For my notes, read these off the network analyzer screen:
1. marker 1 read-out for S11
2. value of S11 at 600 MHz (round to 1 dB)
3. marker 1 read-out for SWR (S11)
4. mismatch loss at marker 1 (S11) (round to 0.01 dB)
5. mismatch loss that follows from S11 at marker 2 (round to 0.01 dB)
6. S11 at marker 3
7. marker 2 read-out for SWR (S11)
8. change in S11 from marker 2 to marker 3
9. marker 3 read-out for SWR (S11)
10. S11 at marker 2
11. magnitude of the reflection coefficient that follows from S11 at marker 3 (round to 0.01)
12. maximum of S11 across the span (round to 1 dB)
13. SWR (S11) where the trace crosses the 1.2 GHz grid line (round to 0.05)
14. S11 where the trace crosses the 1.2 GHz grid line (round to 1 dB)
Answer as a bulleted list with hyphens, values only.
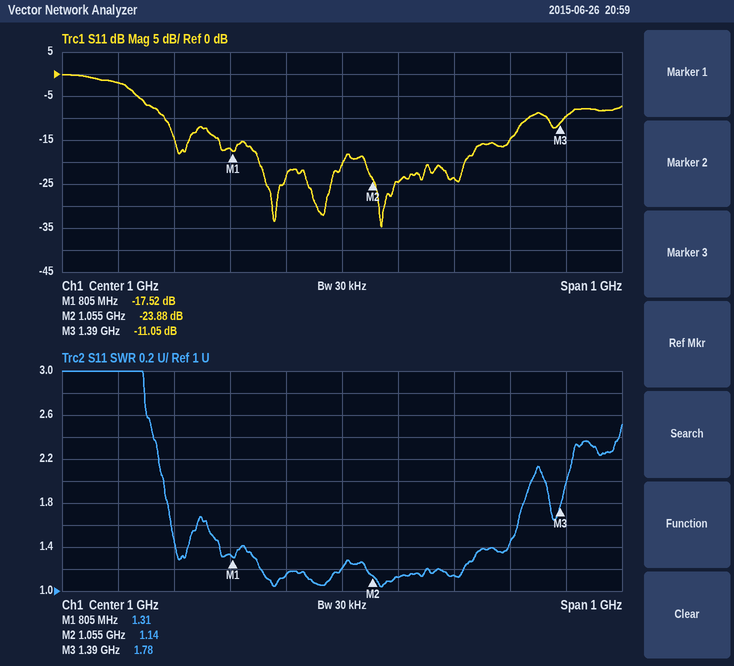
- -17.52 dB
- -2 dB
- 1.31
- 0.08 dB
- 0.02 dB
- -11.05 dB
- 1.14
- 12.83 dB
- 1.78
- -23.88 dB
- 0.28
- 0 dB
- 1.15
- -24 dB
